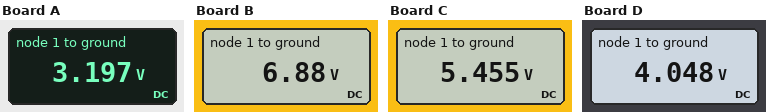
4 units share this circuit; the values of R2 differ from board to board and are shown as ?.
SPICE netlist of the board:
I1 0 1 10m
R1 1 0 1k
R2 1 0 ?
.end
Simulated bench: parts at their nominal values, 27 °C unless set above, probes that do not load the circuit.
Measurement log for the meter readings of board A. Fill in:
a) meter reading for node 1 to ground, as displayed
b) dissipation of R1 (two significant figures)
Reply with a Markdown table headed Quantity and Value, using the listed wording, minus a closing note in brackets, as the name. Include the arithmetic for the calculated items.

| Quantity | Value |
|---|---|
| meter reading for node 1 to ground, as displayed | 3.197 V |
| dissipation of R1 | (3.197 V)^2 / 1 kΩ = 10 mW |
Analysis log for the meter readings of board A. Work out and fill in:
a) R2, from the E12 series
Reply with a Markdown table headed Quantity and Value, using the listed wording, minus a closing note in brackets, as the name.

| Quantity | Value |
|---|---|
| R2, from the E12 series | 470 Ω |
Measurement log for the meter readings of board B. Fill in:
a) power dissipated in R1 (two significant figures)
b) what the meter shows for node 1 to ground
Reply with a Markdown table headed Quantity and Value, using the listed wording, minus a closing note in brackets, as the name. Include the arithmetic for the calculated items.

| Quantity | Value |
|---|---|
| power dissipated in R1 | (6.88 V)^2 / 1 kΩ = 47 mW |
| what the meter shows for node 1 to ground | 6.88 V |
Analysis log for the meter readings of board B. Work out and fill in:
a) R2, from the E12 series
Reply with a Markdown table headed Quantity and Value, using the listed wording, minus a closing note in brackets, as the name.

| Quantity | Value |
|---|---|
| R2, from the E12 series | 2.2 kΩ |
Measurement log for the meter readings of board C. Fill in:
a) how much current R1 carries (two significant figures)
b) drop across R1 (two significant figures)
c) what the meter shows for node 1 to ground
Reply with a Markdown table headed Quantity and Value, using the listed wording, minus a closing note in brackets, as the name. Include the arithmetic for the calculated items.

| Quantity | Value |
|---|---|
| how much current R1 carries | (5.455 V) / 1 kΩ = 5.5 mA |
| drop across R1 | 5.455 V = 5.5 V |
| what the meter shows for node 1 to ground | 5.455 V |
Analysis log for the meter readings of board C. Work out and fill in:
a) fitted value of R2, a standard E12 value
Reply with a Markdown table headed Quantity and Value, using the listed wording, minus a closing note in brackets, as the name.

| Quantity | Value |
|---|---|
| fitted value of R2, a standard E12 value | 1.2 kΩ |
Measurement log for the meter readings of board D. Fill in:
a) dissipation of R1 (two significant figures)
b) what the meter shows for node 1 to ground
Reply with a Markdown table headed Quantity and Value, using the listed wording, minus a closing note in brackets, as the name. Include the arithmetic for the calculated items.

| Quantity | Value |
|---|---|
| dissipation of R1 | (4.048 V)^2 / 1 kΩ = 16 mW |
| what the meter shows for node 1 to ground | 4.048 V |
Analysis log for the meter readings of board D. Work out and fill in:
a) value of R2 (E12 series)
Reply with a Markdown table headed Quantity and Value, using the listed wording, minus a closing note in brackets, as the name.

| Quantity | Value |
|---|---|
| value of R2 | 680 Ω |
